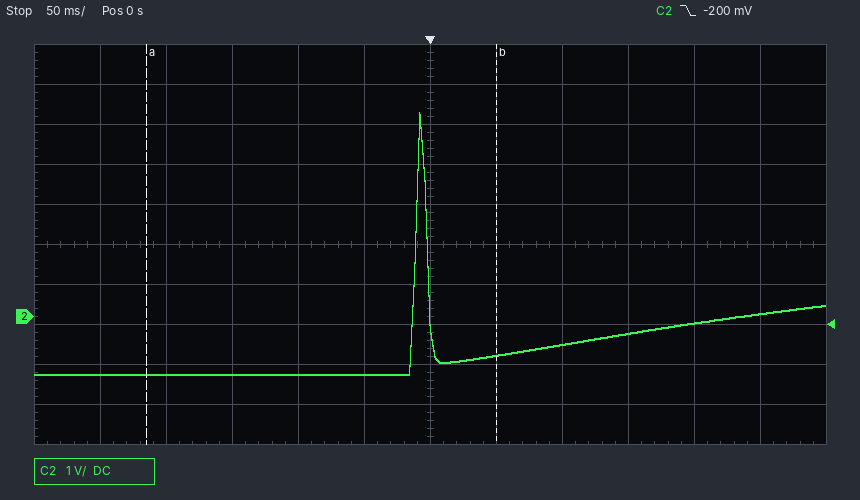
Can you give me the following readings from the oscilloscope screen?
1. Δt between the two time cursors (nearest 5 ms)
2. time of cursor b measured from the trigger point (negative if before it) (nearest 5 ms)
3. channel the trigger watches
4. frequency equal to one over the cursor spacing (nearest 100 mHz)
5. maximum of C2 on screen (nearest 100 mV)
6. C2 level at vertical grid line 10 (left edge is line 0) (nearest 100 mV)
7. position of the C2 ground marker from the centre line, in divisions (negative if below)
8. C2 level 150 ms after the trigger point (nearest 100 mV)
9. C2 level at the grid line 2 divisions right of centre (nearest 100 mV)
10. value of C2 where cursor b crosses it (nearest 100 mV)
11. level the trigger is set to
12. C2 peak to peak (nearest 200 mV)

265 ms
+50 ms
C2
3.8 Hz
5.1 V
-200 mV
-1.8 div
-400 mV
-700 mV
-1.0 V
-200 mV
6.6 V
